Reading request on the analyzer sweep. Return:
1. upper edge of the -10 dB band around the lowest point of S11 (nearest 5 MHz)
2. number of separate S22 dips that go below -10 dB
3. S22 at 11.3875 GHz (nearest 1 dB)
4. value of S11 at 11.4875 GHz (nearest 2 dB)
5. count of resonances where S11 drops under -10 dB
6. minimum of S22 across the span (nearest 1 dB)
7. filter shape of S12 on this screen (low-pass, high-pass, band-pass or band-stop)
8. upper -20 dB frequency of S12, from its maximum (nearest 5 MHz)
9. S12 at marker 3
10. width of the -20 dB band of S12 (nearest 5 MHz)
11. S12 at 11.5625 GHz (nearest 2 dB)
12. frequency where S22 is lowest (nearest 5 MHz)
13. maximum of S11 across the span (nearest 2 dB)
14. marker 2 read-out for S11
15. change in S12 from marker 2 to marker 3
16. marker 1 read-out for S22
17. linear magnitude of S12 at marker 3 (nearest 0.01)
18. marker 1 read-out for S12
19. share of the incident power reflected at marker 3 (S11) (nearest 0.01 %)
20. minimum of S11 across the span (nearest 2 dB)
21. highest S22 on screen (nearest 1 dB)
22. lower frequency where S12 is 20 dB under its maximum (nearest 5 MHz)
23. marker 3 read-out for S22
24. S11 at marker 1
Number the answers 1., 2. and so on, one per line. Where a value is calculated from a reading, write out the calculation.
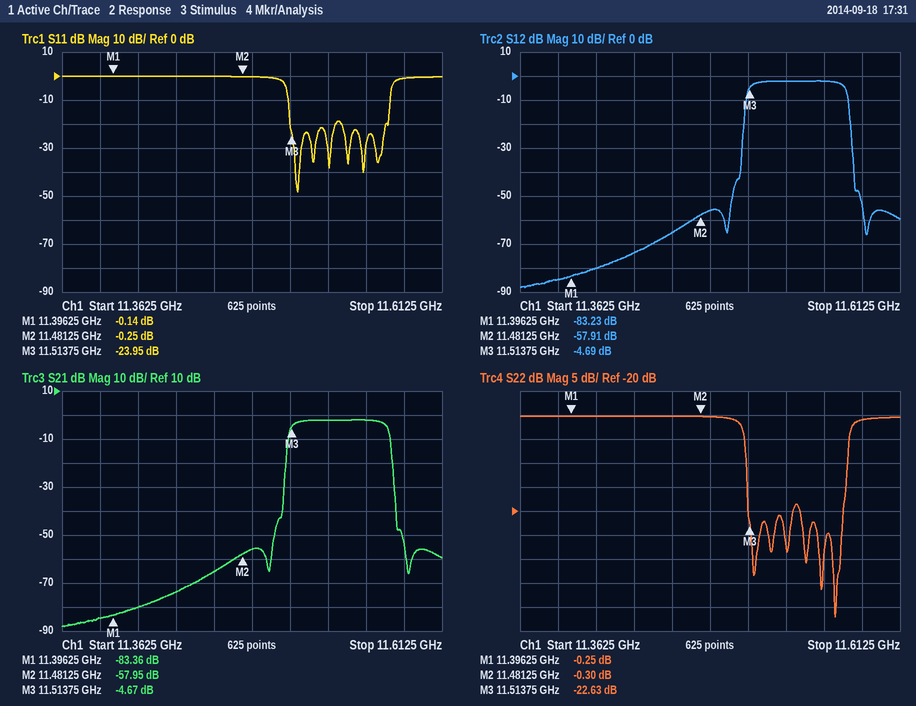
1. 11.580 GHz
2. 6
3. 0 dB
4. 0 dB
5. 6
6. -42 dB
7. band-pass
8. 11.580 GHz
9. -4.69 dB
10. 11.580 GHz − 11.510 GHz = 70 MHz
11. -2 dB
12. 11.570 GHz
13. 0 dB
14. -0.25 dB
15. -4.69 − (-57.91) = 53.22 dB
16. -0.25 dB
17. 10^(-4.69/20) ≈ 0.58
18. -83.23 dB
19. 10^(-23.95/10) ≈ 0.40 %
20. -48 dB
21. 0 dB
22. 11.510 GHz
23. -22.63 dB
24. -0.14 dB
